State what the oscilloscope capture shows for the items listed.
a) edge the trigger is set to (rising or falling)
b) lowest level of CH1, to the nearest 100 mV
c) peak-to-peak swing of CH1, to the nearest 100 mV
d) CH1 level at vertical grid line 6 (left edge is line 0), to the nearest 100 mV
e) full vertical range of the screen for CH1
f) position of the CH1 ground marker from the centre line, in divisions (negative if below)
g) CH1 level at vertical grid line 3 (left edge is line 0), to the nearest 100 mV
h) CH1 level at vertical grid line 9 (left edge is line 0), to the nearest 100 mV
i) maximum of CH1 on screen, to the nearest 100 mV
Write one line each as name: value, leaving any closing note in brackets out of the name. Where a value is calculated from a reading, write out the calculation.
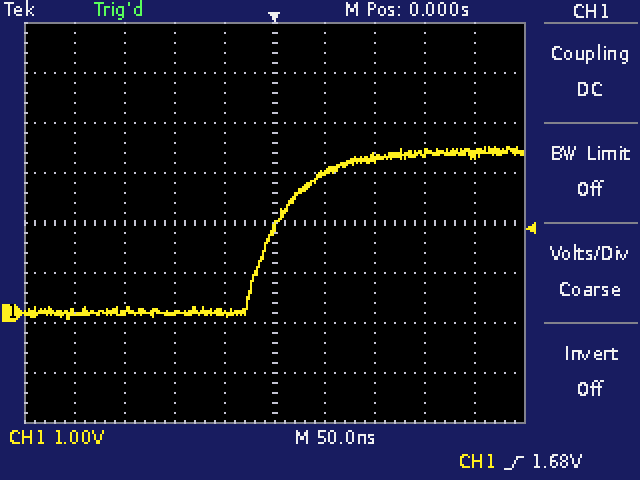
edge the trigger is set to: rising
lowest level of CH1, to the nearest 100 mV: -100 mV
peak-to-peak swing of CH1, to the nearest 100 mV: 3.3 V − (-100 mV) = 3.4 V
CH1 level at vertical grid line 6 (left edge is line 0), to the nearest 100 mV: 2.8 V
full vertical range of the screen for CH1: 8 V
position of the CH1 ground marker from the centre line, in divisions: -1.8 div
CH1 level at vertical grid line 3 (left edge is line 0), to the nearest 100 mV: 0.0 V
CH1 level at vertical grid line 9 (left edge is line 0), to the nearest 100 mV: 3.2 V
maximum of CH1 on screen, to the nearest 100 mV: 3.3 V
